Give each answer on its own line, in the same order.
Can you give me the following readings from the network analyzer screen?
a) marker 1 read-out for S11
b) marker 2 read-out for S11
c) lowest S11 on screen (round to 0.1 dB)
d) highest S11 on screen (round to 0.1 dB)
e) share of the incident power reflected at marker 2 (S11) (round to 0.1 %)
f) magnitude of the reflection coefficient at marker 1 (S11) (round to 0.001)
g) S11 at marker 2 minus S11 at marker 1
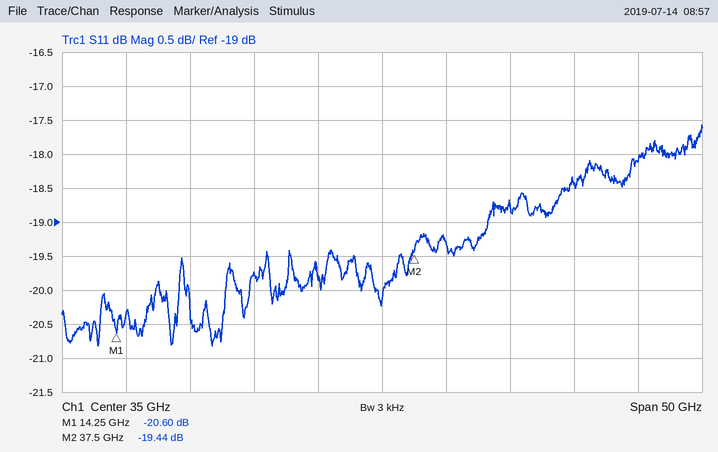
-20.60 dB
-19.44 dB
-20.8 dB
-17.6 dB
1.1 %
0.093
1.16 dB
